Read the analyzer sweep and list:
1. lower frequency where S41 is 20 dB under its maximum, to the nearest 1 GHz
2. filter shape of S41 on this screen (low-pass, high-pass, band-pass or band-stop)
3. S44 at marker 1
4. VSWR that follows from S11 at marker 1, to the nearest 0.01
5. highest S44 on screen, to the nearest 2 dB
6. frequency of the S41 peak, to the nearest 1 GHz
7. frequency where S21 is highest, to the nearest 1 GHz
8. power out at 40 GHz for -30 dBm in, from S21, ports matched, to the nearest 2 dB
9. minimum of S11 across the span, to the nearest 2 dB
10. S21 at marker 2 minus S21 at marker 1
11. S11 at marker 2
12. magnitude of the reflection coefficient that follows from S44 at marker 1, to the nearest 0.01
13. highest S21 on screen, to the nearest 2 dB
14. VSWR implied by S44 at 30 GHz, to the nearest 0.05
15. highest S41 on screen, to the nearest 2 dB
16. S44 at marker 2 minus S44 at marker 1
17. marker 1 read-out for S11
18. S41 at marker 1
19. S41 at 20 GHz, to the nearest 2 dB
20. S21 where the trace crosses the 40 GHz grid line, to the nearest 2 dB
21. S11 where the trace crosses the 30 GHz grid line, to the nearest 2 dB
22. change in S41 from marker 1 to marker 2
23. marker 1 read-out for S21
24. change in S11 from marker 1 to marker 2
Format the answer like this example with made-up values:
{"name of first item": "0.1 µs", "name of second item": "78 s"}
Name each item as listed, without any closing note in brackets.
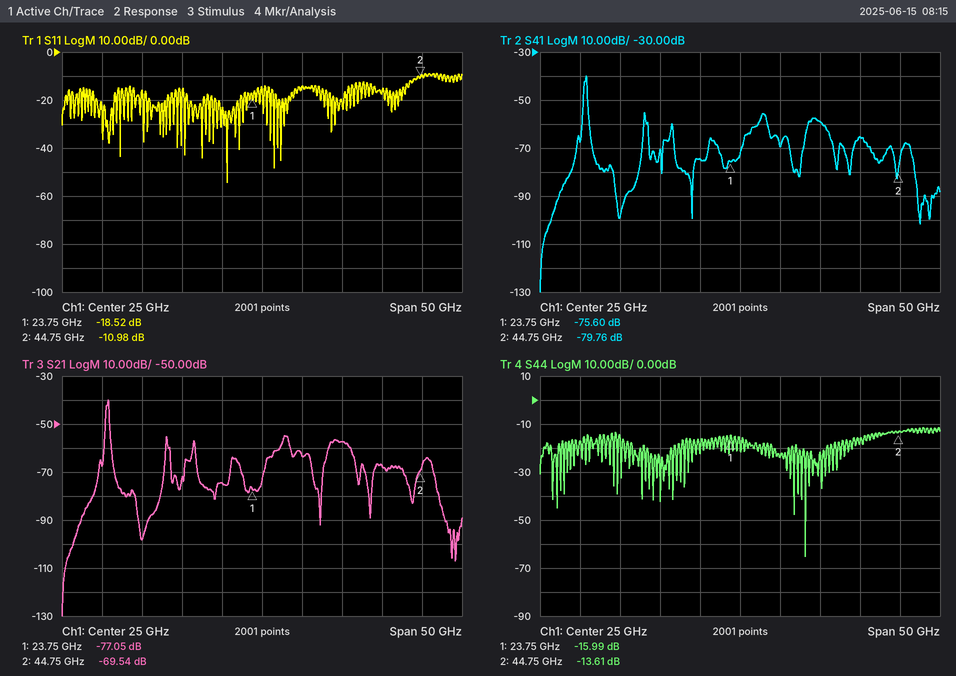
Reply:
{"lower frequency where S41 is 20 dB under its maximum, to the nearest 1 GHz": "5 GHz", "filter shape of S41 on this screen": "band-pass", "S44 at marker 1": "-15.99 dB", "VSWR that follows from S11 at marker 1, to the nearest 0.01": "1.27", "highest S44 on screen, to the nearest 2 dB": "-12 dB", "frequency of the S41 peak, to the nearest 1 GHz": "6 GHz", "frequency where S21 is highest, to the nearest 1 GHz": "6 GHz", "power out at 40 GHz for -30 dBm in, from S21, ports matched, to the nearest 2 dB": "-98 dBm", "minimum of S11 across the span, to the nearest 2 dB": "-54 dB", "S21 at marker 2 minus S21 at marker 1": "7.51 dB", "S11 at marker 2": "-10.98 dB", "magnitude of the reflection coefficient that follows from S44 at marker 1, to the nearest 0.01": "0.16", "highest S21 on screen, to the nearest 2 dB": "-40 dB", "VSWR implied by S44 at 30 GHz, to the nearest 0.05": "1.15", "highest S41 on screen, to the nearest 2 dB": "-40 dB", "S44 at marker 2 minus S44 at marker 1": "2.38 dB", "marker 1 read-out for S11": "-18.52 dB", "S41 at marker 1": "-75.60 dB", "S41 at 20 GHz, to the nearest 2 dB": "-74 dB", "S21 where the trace crosses the 40 GHz grid line, to the nearest 2 dB": "-68 dB", "S11 where the trace crosses the 30 GHz grid line, to the nearest 2 dB": "-14 dB", "change in S41 from marker 1 to marker 2": "-4.16 dB", "marker 1 read-out for S21": "-77.05 dB", "change in S11 from marker 1 to marker 2": "7.54 dB"}
